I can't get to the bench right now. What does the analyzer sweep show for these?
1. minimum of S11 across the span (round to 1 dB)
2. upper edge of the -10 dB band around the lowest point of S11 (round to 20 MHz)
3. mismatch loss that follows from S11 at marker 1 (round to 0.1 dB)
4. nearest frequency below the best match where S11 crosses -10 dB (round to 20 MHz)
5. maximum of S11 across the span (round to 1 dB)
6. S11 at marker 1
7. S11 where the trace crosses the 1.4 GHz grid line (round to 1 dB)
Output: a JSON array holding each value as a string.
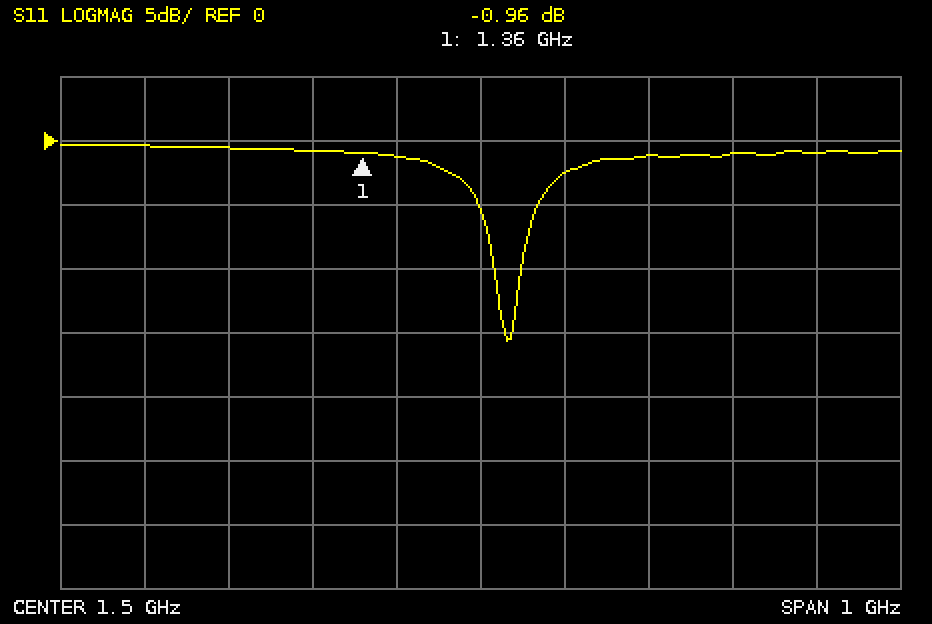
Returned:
["-16 dB", "1.54 GHz", "7.0 dB", "1.52 GHz", "0 dB", "-0.96 dB", "-1 dB"]
